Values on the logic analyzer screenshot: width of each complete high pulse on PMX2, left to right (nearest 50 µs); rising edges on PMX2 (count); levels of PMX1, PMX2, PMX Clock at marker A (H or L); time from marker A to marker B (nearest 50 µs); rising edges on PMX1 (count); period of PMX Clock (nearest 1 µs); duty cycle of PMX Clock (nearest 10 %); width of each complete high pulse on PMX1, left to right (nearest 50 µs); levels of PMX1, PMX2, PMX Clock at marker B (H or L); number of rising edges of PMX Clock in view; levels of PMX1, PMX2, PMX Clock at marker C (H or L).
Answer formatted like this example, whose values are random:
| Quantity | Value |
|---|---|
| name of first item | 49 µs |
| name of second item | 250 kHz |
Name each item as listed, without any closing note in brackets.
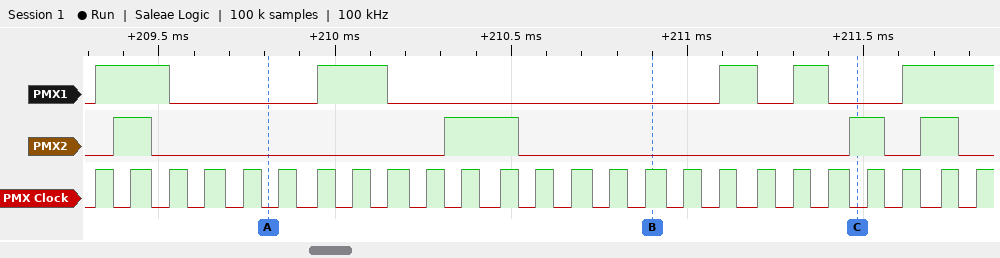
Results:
| Quantity | Value |
|---|---|
| width of each complete high pulse on PMX2, left to right | 100 µs, 200 µs, 100 µs, 100 µs |
| rising edges on PMX2 | 4 |
| levels of PMX1, PMX2, PMX Clock at marker A | PMX1=L, PMX2=L, PMX Clock=L |
| time from marker A to marker B | 1100 µs |
| rising edges on PMX1 | 5 |
| period of PMX Clock | 104 µs |
| duty cycle of PMX Clock | 50 % |
| width of each complete high pulse on PMX1, left to right | 200 µs, 200 µs, 100 µs, 100 µs |
| levels of PMX1, PMX2, PMX Clock at marker B | PMX1=L, PMX2=L, PMX Clock=H |
| number of rising edges of PMX Clock in view | 25 |
| levels of PMX1, PMX2, PMX Clock at marker C | PMX1=L, PMX2=H, PMX Clock=L |
